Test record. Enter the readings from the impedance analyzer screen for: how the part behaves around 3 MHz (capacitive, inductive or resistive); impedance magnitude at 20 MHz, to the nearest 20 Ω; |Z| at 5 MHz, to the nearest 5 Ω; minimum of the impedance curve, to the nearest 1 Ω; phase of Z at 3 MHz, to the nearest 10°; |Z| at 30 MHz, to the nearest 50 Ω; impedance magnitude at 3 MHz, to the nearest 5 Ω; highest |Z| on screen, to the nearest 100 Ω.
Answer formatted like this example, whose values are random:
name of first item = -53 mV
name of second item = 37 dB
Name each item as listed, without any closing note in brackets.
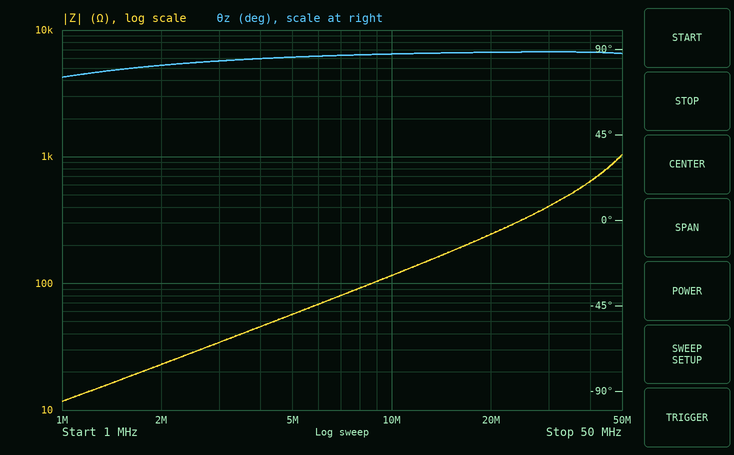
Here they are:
how the part behaves around 3 MHz = inductive
impedance magnitude at 20 MHz, to the nearest 20 Ω = 240 Ω
|Z| at 5 MHz, to the nearest 5 Ω = 55 Ω
minimum of the impedance curve, to the nearest 1 Ω = 12 Ω
phase of Z at 3 MHz, to the nearest 10° = 80°
|Z| at 30 MHz, to the nearest 50 Ω = 400 Ω
impedance magnitude at 3 MHz, to the nearest 5 Ω = 35 Ω
highest |Z| on screen, to the nearest 100 Ω = 1.0 kΩ
